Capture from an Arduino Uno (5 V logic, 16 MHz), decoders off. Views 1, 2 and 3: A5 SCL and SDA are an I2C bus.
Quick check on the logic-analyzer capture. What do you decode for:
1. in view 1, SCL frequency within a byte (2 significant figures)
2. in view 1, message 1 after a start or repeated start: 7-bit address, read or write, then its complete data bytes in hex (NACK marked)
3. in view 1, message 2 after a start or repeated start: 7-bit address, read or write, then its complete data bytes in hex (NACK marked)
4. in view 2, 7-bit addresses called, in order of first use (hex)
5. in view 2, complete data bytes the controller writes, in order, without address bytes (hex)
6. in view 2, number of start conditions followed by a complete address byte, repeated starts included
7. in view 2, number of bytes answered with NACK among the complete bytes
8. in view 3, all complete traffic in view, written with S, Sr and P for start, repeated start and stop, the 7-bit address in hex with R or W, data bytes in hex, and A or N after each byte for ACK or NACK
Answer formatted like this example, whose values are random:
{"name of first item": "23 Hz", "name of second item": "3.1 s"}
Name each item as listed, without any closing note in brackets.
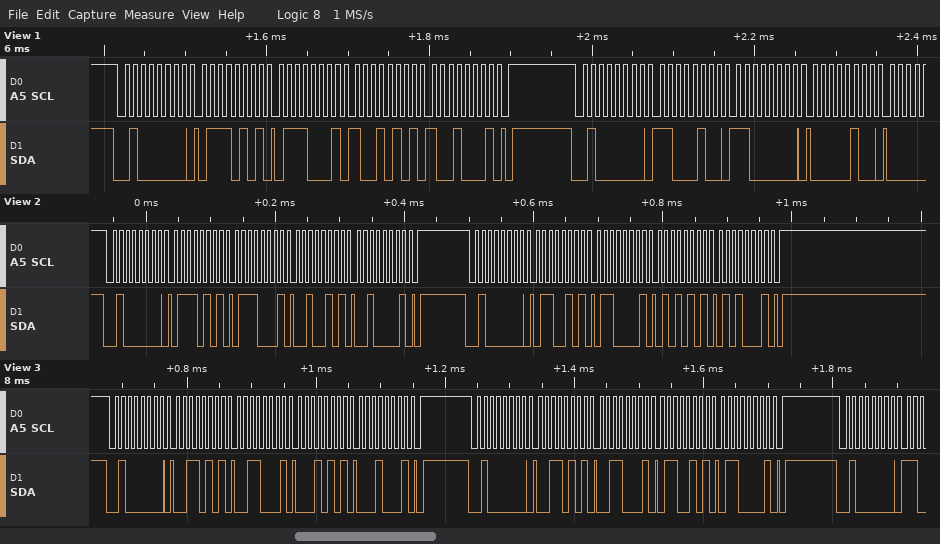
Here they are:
{"in view 1, SCL frequency within a byte": "100 kHz", "in view 1, message 1 after a start or repeated start: 7-bit address, read or write, then its complete data bytes in hex": "0x20 write: 75 71 95 91", "in view 1, message 2 after a start or repeated start: 7-bit address, read or write, then its complete data bytes in hex": "0x20 write: C4 C0 04", "in view 2, 7-bit addresses called, in order of first use": "0x20", "in view 2, complete data bytes the controller writes, in order, without address bytes": "75 71 25 21 65 61 55 51", "in view 2, number of start conditions followed by a complete address byte, repeated starts included": "2", "in view 2, number of bytes answered with NACK among the complete bytes": "0", "in view 3, all complete traffic in view, written with S, Sr and P for start, repeated start and stop, the 7-bit address in hex with R or W, data bytes in hex, and A or N after each byte for ACK or NACK": "S 20W A 35 A 31 A 15 A 11 A P S 20W A 35 A 31 A 65 A 61 A P S 20W A"}
